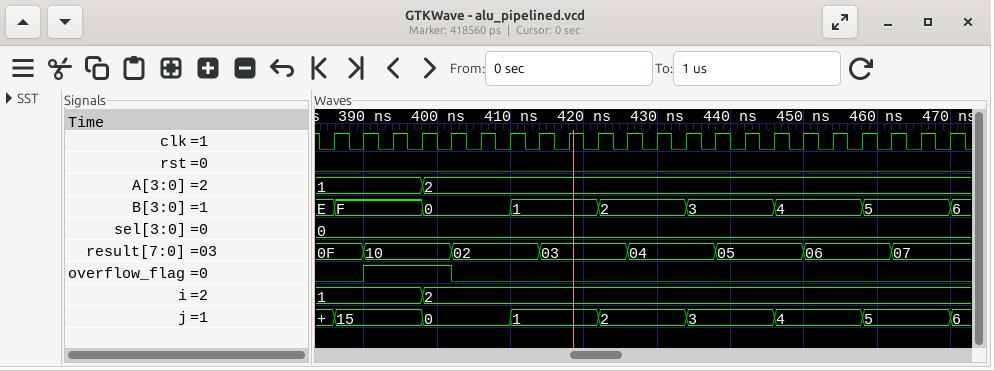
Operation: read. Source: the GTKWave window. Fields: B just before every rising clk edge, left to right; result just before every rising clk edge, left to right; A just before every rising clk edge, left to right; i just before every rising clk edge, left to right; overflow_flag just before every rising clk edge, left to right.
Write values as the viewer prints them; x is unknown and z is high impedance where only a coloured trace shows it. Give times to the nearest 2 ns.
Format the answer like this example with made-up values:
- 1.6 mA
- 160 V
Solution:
- E, F, F, F, 0, 0, 0, 1, 1, 1, 2, 2, 2, 3, 3, 3, 4, 4, 4, 5, 5, 5
- 0F, 0F, 10, 10, 10, 02, 02, 02, 03, 03, 03, 04, 04, 04, 05, 05, 05, 06, 06, 06, 07, 07
- 1, 1, 1, 1, 2, 2, 2, 2, 2, 2, 2, 2, 2, 2, 2, 2, 2, 2, 2, 2, 2, 2
- 1, 1, 1, 1, 2, 2, 2, 2, 2, 2, 2, 2, 2, 2, 2, 2, 2, 2, 2, 2, 2, 2
- 0 0 1 1 1 0 0 0 0 0 0 0 0 0 0 0 0 0 0 0 0 0
